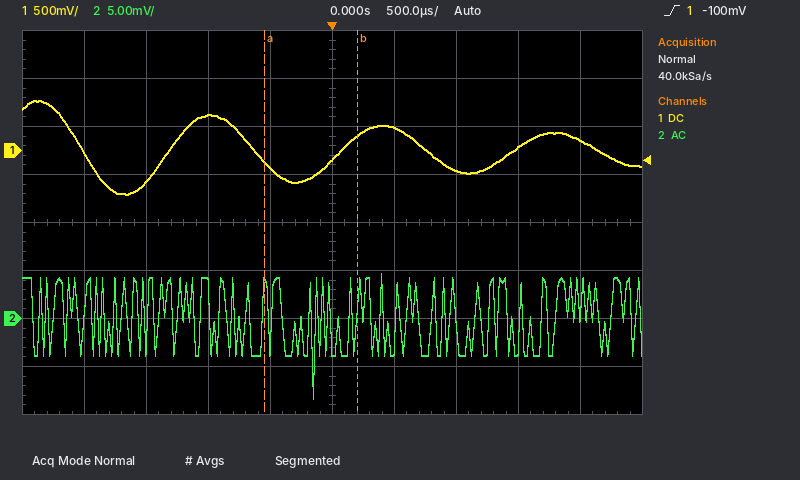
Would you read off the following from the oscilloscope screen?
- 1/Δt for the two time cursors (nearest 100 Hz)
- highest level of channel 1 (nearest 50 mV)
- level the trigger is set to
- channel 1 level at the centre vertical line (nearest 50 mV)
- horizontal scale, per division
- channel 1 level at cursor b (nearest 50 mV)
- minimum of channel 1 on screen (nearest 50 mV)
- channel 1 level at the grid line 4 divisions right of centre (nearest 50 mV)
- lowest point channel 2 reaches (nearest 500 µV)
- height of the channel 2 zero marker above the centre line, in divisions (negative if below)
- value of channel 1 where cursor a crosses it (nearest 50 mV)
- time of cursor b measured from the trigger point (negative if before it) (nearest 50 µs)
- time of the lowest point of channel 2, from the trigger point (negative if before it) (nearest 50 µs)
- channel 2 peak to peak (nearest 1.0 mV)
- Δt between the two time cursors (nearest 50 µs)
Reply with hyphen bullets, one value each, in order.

- 1.3 kHz
- 500 mV
- -100 mV
- -100 mV
- 500 µs
- 150 mV
- -450 mV
- 100 mV
- -8.5 mV
- -2.0 div
- -100 mV
- +200 µs
- -150 µs
- 13.0 mV
- 750 µs
